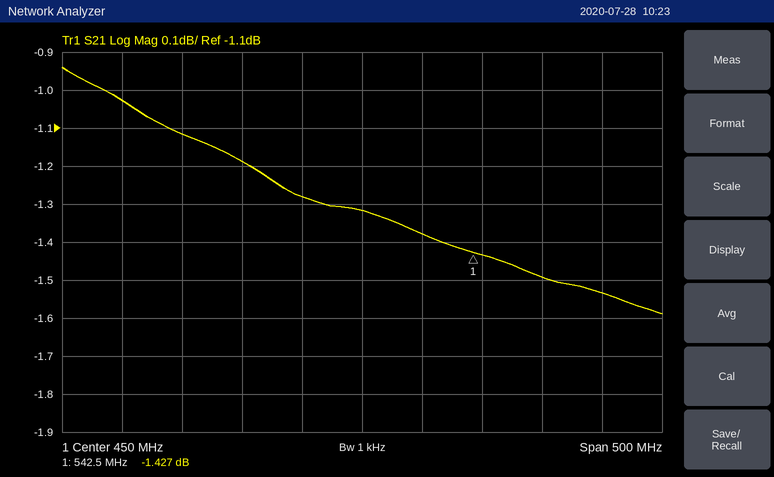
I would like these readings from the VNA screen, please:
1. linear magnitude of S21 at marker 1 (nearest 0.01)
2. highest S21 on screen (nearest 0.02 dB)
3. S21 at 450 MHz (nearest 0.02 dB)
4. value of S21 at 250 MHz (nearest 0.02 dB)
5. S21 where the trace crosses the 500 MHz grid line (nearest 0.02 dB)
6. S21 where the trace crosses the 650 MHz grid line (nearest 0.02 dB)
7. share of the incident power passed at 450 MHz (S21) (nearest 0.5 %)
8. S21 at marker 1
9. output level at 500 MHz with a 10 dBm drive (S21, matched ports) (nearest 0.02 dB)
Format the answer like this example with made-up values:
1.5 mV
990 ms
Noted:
0.85
-0.94 dB
-1.32 dB
-1.02 dB
-1.38 dB
-1.54 dB
74.0 %
-1.427 dB
8.62 dBm
